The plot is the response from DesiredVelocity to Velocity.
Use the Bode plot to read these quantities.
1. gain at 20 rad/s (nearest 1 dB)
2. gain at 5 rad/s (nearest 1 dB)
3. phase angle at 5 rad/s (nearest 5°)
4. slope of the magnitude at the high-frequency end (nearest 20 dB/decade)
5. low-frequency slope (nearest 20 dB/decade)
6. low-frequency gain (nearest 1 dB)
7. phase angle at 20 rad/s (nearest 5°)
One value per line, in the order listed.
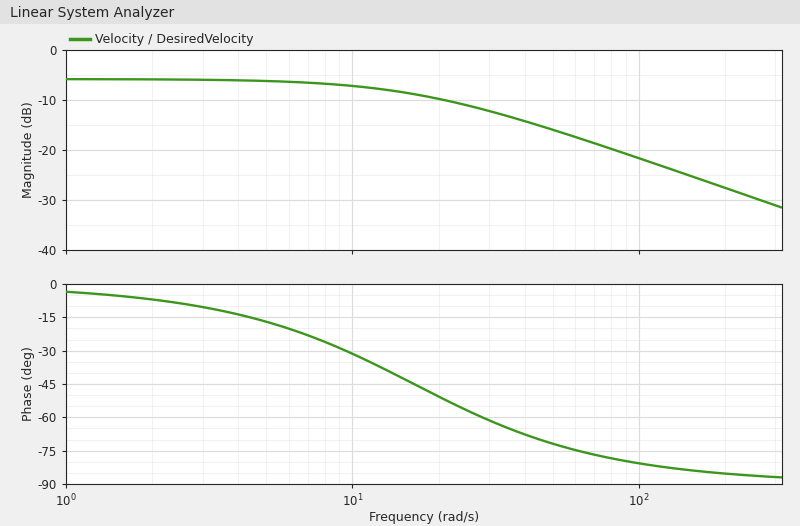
-10 dB
-6 dB
-15°
-20 dB/decade
0 dB/decade
-6 dB
-50°
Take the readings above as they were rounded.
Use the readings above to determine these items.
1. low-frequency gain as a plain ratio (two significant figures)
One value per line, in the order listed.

0.50
